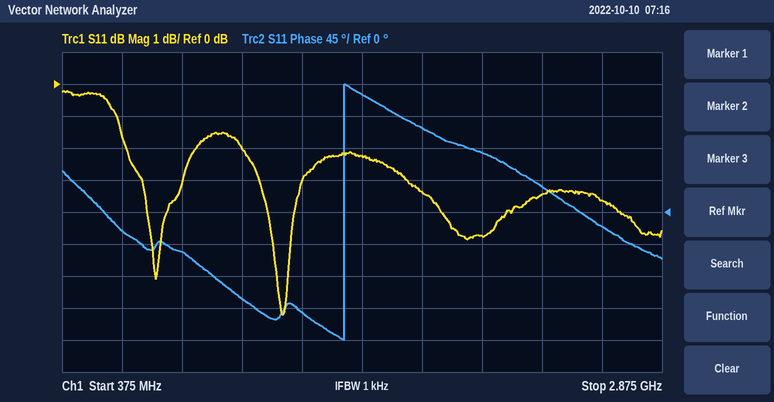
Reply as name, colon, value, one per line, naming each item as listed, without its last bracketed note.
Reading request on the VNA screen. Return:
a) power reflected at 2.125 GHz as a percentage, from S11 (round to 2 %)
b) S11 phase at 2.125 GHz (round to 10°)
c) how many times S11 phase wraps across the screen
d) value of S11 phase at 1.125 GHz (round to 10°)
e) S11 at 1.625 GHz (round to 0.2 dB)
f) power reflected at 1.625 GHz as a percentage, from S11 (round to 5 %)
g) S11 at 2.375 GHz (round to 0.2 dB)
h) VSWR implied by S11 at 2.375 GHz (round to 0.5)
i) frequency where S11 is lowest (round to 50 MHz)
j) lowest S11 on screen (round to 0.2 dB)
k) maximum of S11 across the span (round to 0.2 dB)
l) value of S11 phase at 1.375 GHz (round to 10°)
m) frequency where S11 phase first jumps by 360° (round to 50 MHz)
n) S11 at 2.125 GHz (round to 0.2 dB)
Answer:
power reflected at 2.125 GHz as a percentage, from S11: 34 %
S11 phase at 2.125 GHz: 80°
how many times S11 phase wraps across the screen: 1
value of S11 phase at 1.125 GHz: -120°
S11 at 1.625 GHz: -2.2 dB
power reflected at 1.625 GHz as a percentage, from S11: 60 %
S11 at 2.375 GHz: -3.4 dB
VSWR implied by S11 at 2.375 GHz: 5.0
frequency where S11 is lowest: 1.30 GHz
lowest S11 on screen: -7.2 dB
maximum of S11 across the span: -0.2 dB
value of S11 phase at 1.375 GHz: -140°
frequency where S11 phase first jumps by 360°: 1.55 GHz
S11 at 2.125 GHz: -4.8 dB
